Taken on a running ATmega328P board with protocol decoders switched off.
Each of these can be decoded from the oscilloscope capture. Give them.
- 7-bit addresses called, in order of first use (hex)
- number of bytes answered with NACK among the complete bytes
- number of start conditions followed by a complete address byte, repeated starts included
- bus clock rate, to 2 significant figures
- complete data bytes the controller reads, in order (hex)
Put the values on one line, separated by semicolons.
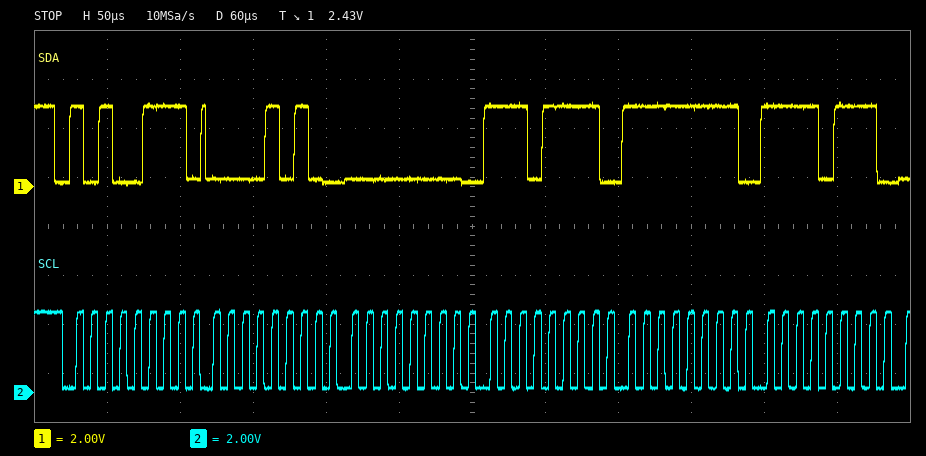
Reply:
0x53; 0; 1; 100 kHz; 0A 00 EF FF F7
